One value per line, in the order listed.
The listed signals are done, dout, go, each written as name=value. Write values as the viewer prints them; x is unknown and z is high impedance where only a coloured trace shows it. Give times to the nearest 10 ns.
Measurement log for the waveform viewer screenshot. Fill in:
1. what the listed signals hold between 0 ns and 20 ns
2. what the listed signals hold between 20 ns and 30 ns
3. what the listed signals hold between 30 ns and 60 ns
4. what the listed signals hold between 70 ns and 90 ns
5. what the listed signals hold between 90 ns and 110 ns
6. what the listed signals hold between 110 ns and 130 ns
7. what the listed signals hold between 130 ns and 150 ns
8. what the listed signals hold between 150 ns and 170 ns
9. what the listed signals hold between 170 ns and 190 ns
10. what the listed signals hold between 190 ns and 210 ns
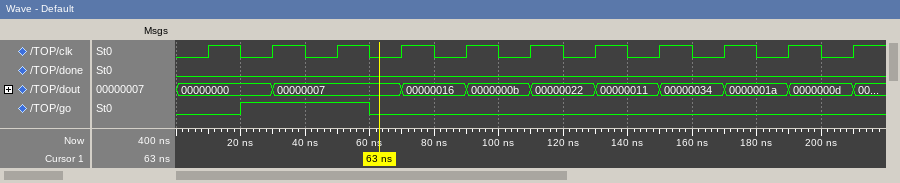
done=0, dout=00000000, go=0
done=0, dout=00000000, go=1
done=0, dout=00000007, go=1
done=0, dout=00000016, go=0
done=0, dout=0000000b, go=0
done=0, dout=00000022, go=0
done=0, dout=00000011, go=0
done=0, dout=00000034, go=0
done=0, dout=0000001a, go=0
done=0, dout=0000000d, go=0
